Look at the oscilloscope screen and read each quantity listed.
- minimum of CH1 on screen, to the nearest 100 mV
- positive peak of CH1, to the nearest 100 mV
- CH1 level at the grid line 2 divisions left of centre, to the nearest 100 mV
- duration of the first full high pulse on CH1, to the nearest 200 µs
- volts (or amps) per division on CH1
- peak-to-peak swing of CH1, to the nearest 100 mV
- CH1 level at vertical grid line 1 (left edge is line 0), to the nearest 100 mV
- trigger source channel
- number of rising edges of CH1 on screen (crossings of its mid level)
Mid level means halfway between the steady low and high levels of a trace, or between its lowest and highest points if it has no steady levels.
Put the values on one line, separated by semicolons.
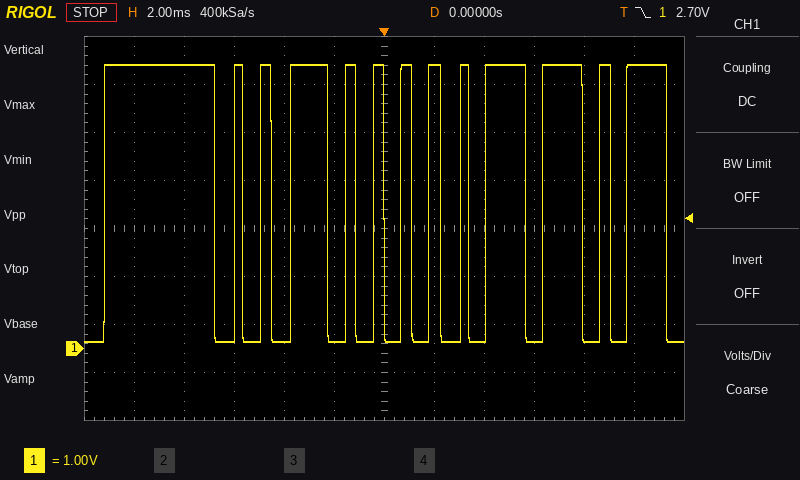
100 mV; 5.9 V; 100 mV; 4.4 ms; 1 V; 5.8 V; 5.9 V; CH1; 13
